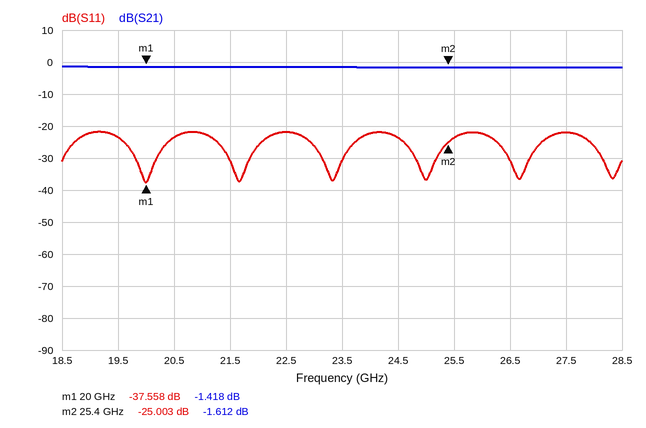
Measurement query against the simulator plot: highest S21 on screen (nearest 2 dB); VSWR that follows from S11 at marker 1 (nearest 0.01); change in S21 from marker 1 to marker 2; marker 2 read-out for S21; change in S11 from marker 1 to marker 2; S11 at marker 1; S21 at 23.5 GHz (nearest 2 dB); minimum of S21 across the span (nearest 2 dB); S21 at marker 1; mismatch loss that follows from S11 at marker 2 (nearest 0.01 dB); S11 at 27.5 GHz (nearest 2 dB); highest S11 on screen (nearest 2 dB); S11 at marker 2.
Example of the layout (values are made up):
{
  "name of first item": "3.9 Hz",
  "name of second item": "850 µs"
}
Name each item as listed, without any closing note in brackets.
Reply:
{
  "highest S21 on screen": "-2 dB",
  "VSWR that follows from S11 at marker 1": "1.03",
  "change in S21 from marker 1 to marker 2": "-0.194 dB",
  "marker 2 read-out for S21": "-1.612 dB",
  "change in S11 from marker 1 to marker 2": "12.555 dB",
  "S11 at marker 1": "-37.558 dB",
  "S21 at 23.5 GHz": "-2 dB",
  "minimum of S21 across the span": "-2 dB",
  "S21 at marker 1": "-1.418 dB",
  "mismatch loss that follows from S11 at marker 2": "0.01 dB",
  "S11 at 27.5 GHz": "-22 dB",
  "highest S11 on screen": "-22 dB",
  "S11 at marker 2": "-25.003 dB"
}
